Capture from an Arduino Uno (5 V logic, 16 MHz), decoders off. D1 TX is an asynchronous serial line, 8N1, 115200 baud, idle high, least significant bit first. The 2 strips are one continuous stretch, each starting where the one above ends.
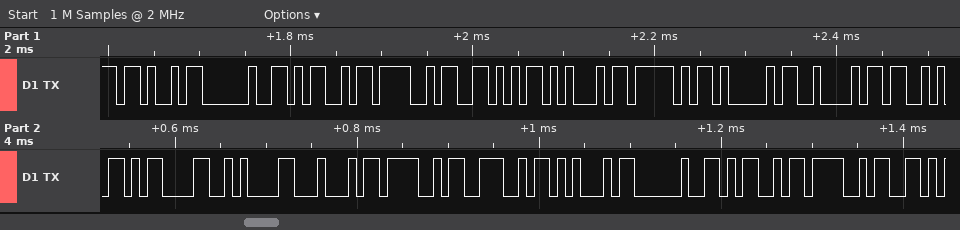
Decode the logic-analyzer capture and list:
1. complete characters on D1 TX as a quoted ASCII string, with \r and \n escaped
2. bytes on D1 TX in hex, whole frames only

"K MOVE_ABS\r\nDONE MO"
0x4B 0x20 0x4D 0x4F 0x56 0x45 0x5F 0x41 0x42 0x53 0x0D 0x0A 0x44 0x4F 0x4E 0x45 0x20 0x4D 0x4F
